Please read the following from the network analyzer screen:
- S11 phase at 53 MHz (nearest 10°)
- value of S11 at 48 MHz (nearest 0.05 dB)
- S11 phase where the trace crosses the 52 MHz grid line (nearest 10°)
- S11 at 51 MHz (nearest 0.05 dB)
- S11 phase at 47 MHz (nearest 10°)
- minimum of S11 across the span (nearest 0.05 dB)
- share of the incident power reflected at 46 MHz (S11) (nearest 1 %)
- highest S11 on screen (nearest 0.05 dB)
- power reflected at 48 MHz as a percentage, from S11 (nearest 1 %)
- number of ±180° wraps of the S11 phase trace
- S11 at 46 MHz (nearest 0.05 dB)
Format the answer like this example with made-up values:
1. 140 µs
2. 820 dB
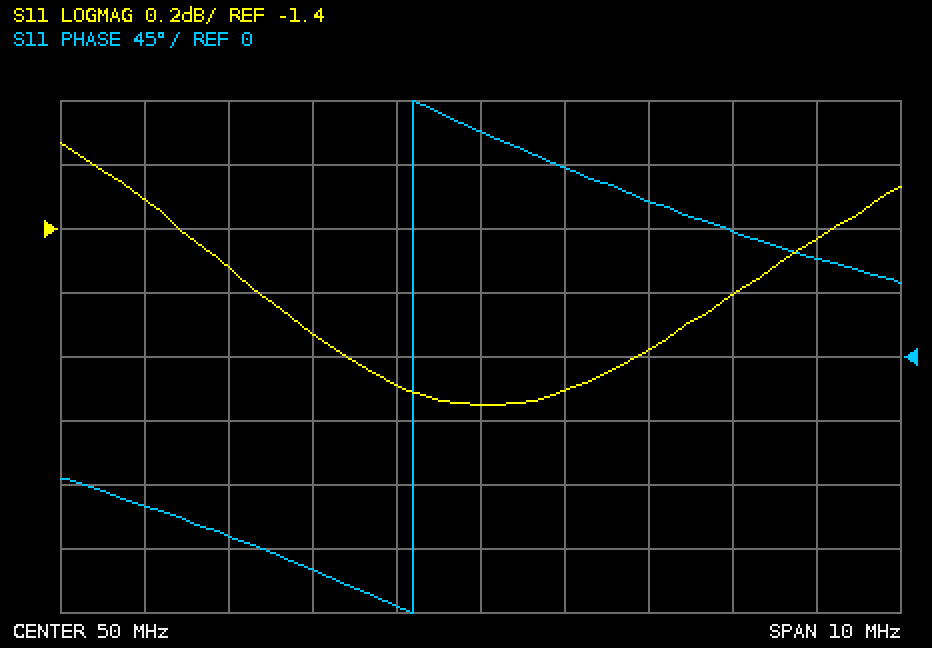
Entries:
1. 90°
2. -1.75 dB
3. 110°
4. -1.90 dB
5. -130°
6. -1.95 dB
7. 74 %
8. -1.15 dB
9. 67 %
10. 1
11. -1.30 dB
